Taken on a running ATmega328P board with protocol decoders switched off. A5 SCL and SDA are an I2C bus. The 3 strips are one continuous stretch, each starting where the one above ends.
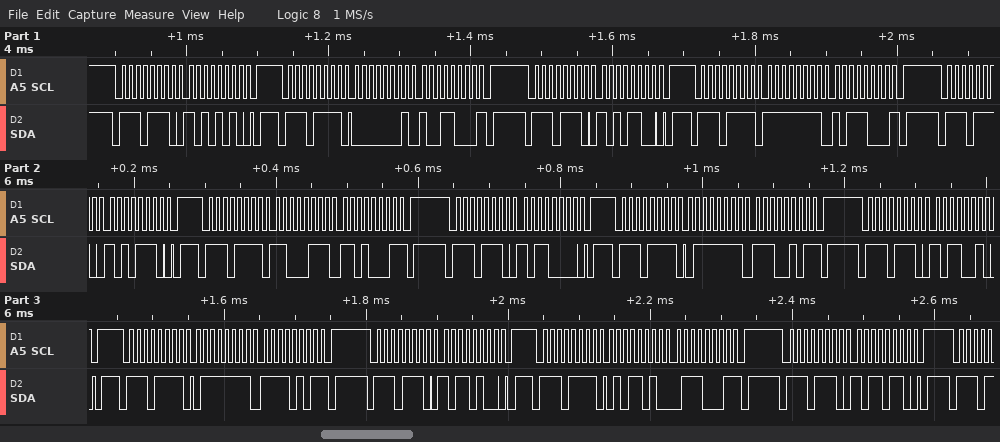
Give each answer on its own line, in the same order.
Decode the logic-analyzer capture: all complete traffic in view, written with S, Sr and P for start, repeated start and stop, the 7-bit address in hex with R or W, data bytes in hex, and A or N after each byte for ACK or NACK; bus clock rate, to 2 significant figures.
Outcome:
S 77W A AA A P S 77R A 01 A 98 N P S 77W A AC A P S 77R A FF A B8 N P S 77W A AE A P S 77R A C7 A D1 N P S 77W A B0 A P S 77R A 7F A E5 N P S 77W A B2 A P S 77R A 7F A F5 N P S 77W A B4 A P S 77R A 5A A 71 N P S 77W A B6 A P
100 kHz
